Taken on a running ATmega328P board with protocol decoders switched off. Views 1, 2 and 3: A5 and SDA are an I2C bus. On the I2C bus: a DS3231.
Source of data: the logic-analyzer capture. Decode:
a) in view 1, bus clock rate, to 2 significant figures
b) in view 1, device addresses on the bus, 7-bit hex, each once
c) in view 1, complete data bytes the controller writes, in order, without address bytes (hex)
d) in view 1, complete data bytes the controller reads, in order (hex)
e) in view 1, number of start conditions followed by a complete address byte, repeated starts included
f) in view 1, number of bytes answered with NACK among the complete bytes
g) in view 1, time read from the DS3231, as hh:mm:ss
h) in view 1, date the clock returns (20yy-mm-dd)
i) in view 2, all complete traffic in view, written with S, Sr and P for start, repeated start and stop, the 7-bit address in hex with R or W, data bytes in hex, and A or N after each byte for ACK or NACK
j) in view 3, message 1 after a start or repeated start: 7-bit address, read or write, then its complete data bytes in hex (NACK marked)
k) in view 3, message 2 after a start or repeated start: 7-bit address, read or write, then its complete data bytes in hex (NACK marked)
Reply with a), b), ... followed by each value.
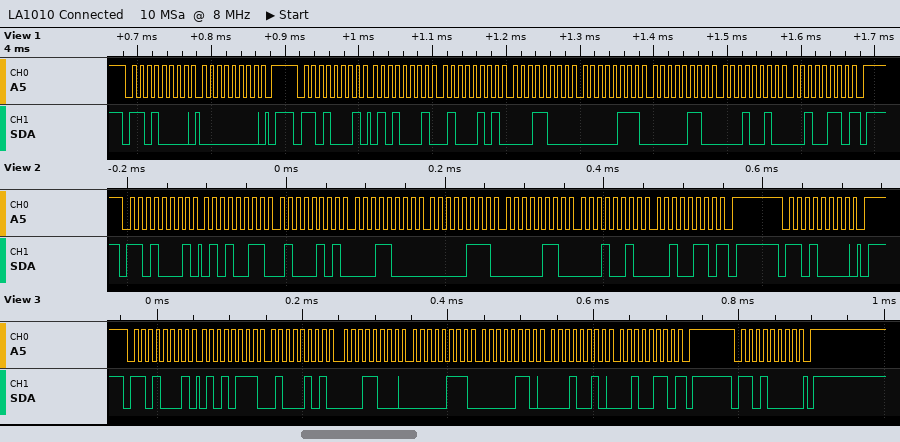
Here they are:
a) 100 kHz
b) 0x68
c) 00
d) 51 45 18 07 06 12 26
e) 2
f) 1
g) 18:45:51
h) 2026-12-06
i) S 68R A 53 A 45 A 18 A 07 A 06 A 12 A 26 N P S 68W A P
j) 0x68 read: 57 45 18 07 06 12 26 NACK
k) 0x68 write
